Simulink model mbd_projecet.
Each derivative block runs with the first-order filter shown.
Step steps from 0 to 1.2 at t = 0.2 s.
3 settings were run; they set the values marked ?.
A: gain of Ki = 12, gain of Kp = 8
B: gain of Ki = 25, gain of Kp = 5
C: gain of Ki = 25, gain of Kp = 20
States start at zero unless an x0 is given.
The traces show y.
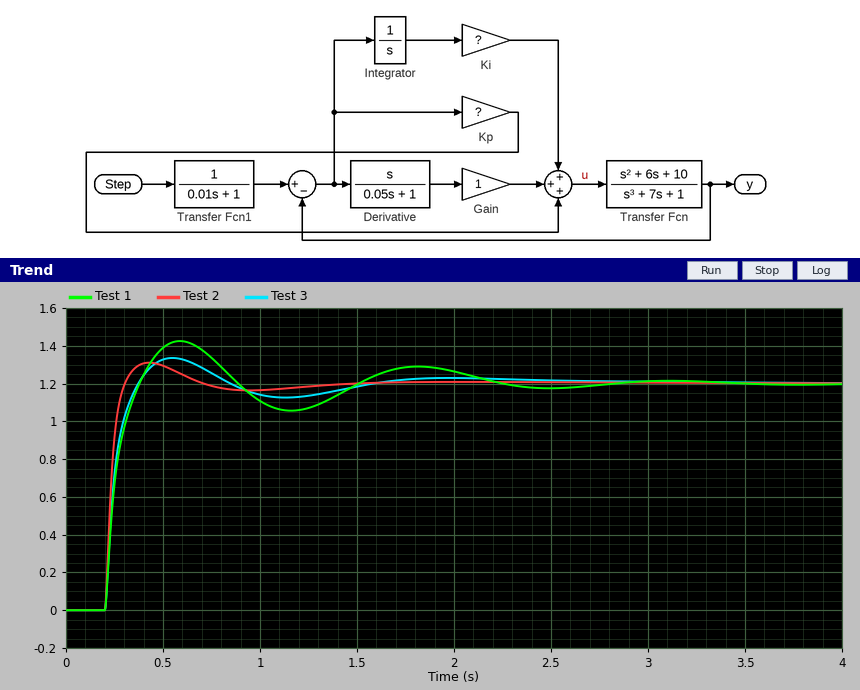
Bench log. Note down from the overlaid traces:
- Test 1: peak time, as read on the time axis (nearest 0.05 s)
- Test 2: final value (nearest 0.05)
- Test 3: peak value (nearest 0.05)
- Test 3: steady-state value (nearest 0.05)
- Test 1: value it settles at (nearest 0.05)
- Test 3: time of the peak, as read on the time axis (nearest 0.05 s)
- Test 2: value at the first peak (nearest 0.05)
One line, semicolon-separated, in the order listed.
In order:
0.60 s; 1.20; 1.35; 1.20; 1.20; 0.55 s; 1.30
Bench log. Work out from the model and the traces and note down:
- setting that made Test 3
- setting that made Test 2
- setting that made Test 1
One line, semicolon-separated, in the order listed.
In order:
A; C; B
